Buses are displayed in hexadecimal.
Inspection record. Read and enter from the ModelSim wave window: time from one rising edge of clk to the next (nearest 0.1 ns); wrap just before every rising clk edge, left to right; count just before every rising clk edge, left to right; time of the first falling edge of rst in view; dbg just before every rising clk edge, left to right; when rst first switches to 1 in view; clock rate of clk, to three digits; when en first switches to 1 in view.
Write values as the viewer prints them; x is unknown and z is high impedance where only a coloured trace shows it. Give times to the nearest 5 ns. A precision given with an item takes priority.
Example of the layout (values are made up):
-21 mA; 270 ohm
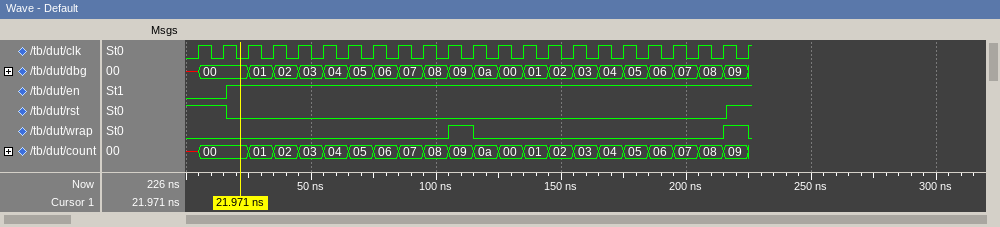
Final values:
10 ns; 0 0 0 0 0 0 0 0 0 0 0 1 0 0 0 0 0 0 0 0 0 0 1; x, 00, 00, 01, 02, 03, 04, 05, 06, 07, 08, 09, 0a, 00, 01, 02, 03, 04, 05, 06, 07, 08, 09; 15 ns; x, 00, 00, 01, 02, 03, 04, 05, 06, 07, 08, 09, 0a, 00, 01, 02, 03, 04, 05, 06, 07, 08, 09; 215 ns; 100 MHz; 15 ns
